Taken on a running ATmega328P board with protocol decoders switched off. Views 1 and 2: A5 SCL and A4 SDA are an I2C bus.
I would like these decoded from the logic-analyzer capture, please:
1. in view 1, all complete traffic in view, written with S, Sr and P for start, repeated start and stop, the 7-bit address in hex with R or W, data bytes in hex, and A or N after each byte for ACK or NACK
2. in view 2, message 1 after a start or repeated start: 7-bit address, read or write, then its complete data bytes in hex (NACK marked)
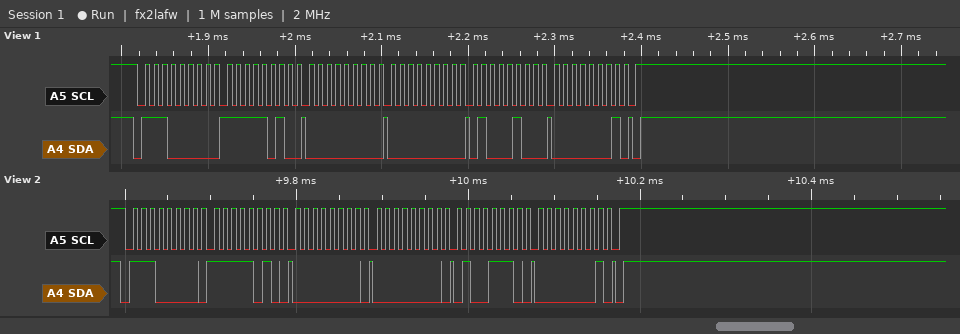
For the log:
S 70W A FA A 00 A 00 A 44 A 01 A P
0x70 write: FA 00 00 4E 01
